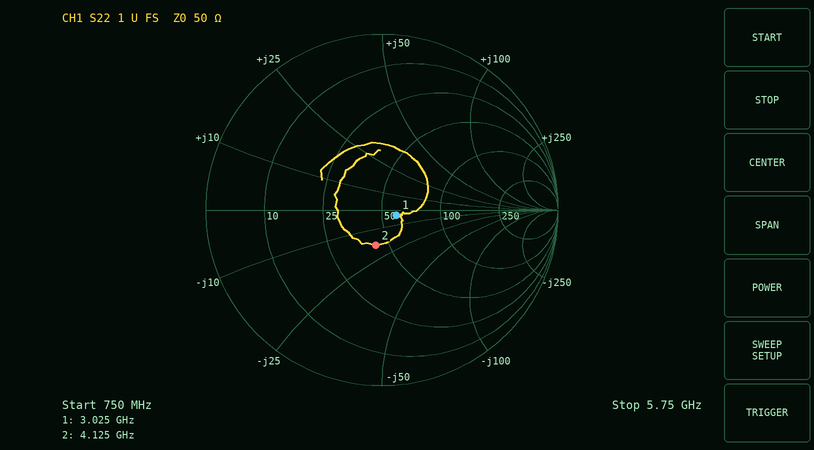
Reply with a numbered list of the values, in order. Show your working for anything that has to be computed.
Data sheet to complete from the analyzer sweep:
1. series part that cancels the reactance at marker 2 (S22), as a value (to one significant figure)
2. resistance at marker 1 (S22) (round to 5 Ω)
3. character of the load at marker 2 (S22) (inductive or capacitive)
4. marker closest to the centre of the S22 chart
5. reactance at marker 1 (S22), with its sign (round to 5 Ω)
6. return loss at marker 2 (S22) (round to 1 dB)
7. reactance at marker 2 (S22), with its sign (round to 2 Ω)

1. L = 18 Ω/(2π × 4.125 GHz) ≈ 694 pH, so 700 pH to one significant figure
2. 60 Ω
3. capacitive
4. marker 1
5. -5 Ω
6. 14 dB
7. -18 Ω
